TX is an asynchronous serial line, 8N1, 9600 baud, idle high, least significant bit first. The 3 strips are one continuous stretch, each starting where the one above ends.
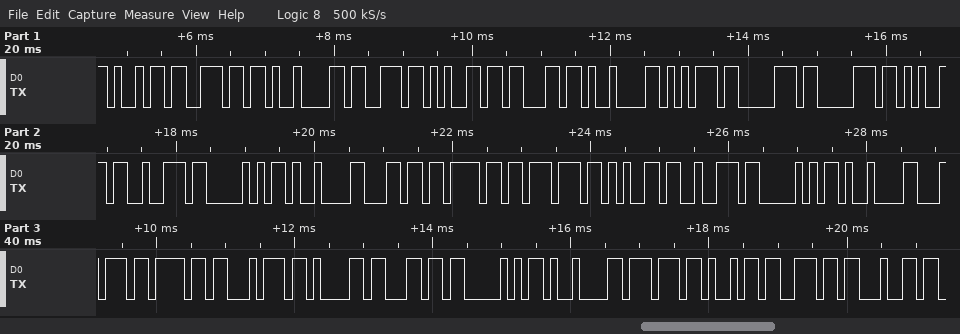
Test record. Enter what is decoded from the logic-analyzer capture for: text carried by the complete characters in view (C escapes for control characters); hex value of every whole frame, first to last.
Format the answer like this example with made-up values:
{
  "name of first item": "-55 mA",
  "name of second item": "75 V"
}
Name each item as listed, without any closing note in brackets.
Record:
{
  "text carried by the complete characters in view": "\"in\\tsec\\tupperP\\tlowerP\\ttotalP\\twind\"",
  "hex value of every whole frame, first to last": "69 6E 09 73 65 63 09 75 70 70 65 72 50 09 6C 6F 77 65 72 50 09 74 6F 74 61 6C 50 09 77 69 6E 64"
}
